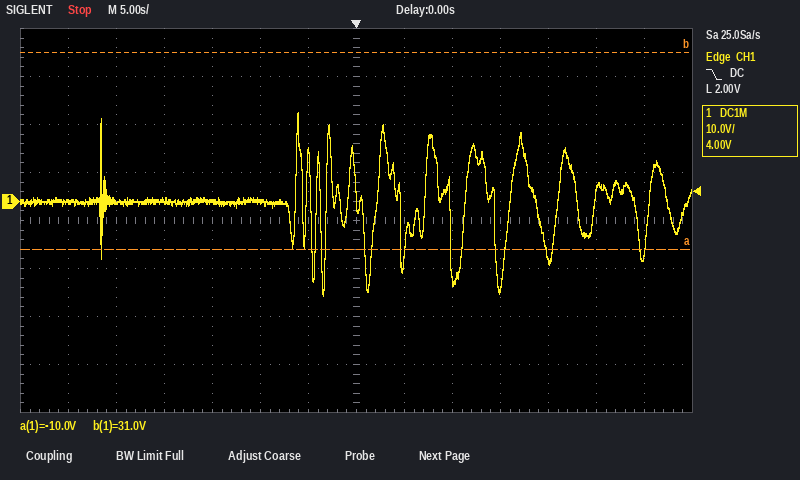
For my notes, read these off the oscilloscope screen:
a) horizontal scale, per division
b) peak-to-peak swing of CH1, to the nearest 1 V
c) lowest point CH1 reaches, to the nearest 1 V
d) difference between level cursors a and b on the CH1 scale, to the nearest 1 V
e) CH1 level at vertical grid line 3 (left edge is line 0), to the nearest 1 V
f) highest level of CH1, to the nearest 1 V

5 s
38 V
-20 V
41 V
0 V
18 V
